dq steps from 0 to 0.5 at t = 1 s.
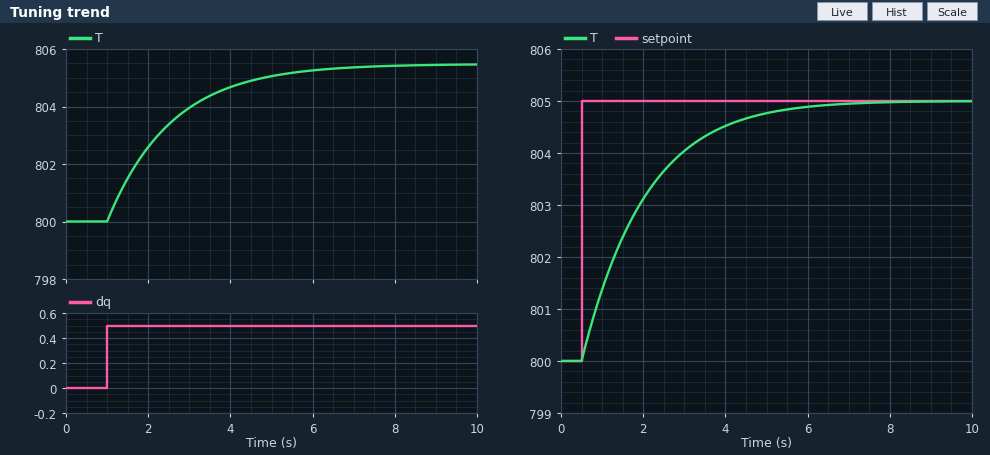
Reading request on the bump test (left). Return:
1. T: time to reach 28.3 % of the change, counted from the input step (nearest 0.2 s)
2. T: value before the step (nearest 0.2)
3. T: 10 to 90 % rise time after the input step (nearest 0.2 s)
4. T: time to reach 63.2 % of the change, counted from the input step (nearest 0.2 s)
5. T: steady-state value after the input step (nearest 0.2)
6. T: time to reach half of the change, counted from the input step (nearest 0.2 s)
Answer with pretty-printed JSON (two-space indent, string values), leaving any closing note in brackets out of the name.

{
  "T: time to reach 28.3 % of the change, counted from the input step": "0.6 s",
  "T: value before the step": "800.0",
  "T: 10 to 90 % rise time after the input step": "3.4 s",
  "T: time to reach 63.2 % of the change, counted from the input step": "1.6 s",
  "T: steady-state value after the input step": "805.4",
  "T: time to reach half of the change, counted from the input step": "1.0 s"
}
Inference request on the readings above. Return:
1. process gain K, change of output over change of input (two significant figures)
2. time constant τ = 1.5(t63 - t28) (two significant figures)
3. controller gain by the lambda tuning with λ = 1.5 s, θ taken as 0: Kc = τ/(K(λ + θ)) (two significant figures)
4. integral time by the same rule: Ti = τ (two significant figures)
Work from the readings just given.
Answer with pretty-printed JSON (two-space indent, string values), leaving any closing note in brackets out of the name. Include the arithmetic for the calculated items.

{
  "process gain K, change of output over change of input": "(805.4 - 800) / 0.5 = 11",
  "time constant τ = 1.5(t63 - t28)": "1.5 × (1.6 - 0.6) = 1.5 s",
  "controller gain by the lambda tuning with λ = 1.5 s, θ taken as 0: Kc = τ/(K(λ + θ))": "1.5 / (11 × (1.5 + 0)) = 0.091",
  "integral time by the same rule: Ti = τ": "1.5 s"
}
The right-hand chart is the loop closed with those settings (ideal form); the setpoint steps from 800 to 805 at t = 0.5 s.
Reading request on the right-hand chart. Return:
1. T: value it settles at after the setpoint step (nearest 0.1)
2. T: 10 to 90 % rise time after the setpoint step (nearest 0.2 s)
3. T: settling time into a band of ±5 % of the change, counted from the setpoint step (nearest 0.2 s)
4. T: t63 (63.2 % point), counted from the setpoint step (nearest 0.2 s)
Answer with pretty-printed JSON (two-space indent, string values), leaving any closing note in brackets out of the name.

{
  "T: value it settles at after the setpoint step": "805.0",
  "T: 10 to 90 % rise time after the setpoint step": "3.2 s",
  "T: settling time into a band of ±5 % of the change, counted from the setpoint step": "4.4 s",
  "T: t63 (63.2 % point), counted from the setpoint step": "1.6 s"
}
